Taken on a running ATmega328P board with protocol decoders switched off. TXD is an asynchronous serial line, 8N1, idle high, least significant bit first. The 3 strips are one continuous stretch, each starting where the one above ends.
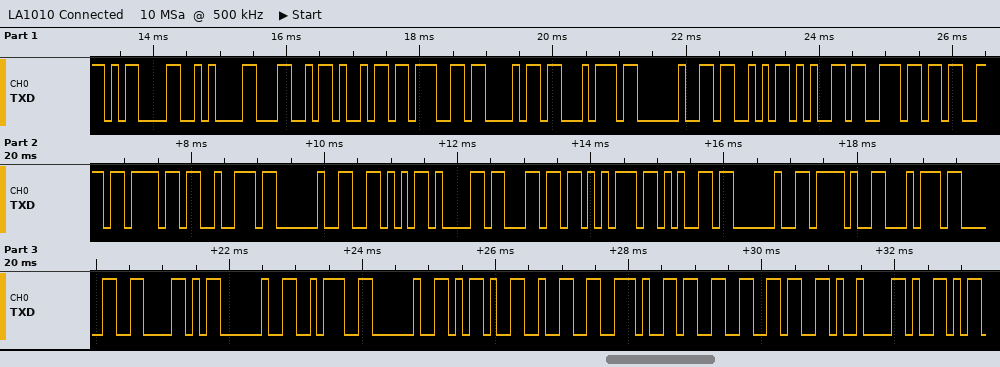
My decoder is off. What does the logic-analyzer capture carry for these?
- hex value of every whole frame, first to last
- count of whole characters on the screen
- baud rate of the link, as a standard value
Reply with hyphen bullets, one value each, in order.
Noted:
- 0D 0A 4C 69 67 68 74 20 53 65 6E 73 6F 72 20 56 61 6C 75 65 20 2F 74 30 58 20 3A 20 2D 32 2E 33 36 09 59
- 35
- 9600 baud
